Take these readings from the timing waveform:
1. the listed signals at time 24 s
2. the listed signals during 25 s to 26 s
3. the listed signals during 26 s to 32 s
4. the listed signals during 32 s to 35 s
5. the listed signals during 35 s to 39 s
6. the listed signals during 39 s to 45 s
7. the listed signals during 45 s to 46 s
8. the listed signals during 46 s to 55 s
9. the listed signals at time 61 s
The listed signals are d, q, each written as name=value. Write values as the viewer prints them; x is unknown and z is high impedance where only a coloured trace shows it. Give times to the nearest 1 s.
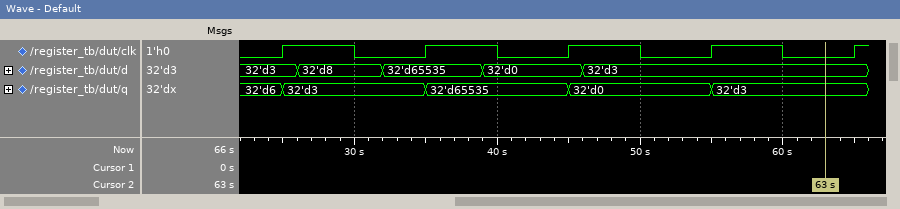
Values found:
d=32'd3, q=32'd6
d=32'd3, q=32'd3
d=32'd8, q=32'd3
d=32'd65535, q=32'd3
d=32'd65535, q=32'd65535
d=32'd0, q=32'd65535
d=32'd0, q=32'd0
d=32'd3, q=32'd0
d=32'd3, q=32'd3
